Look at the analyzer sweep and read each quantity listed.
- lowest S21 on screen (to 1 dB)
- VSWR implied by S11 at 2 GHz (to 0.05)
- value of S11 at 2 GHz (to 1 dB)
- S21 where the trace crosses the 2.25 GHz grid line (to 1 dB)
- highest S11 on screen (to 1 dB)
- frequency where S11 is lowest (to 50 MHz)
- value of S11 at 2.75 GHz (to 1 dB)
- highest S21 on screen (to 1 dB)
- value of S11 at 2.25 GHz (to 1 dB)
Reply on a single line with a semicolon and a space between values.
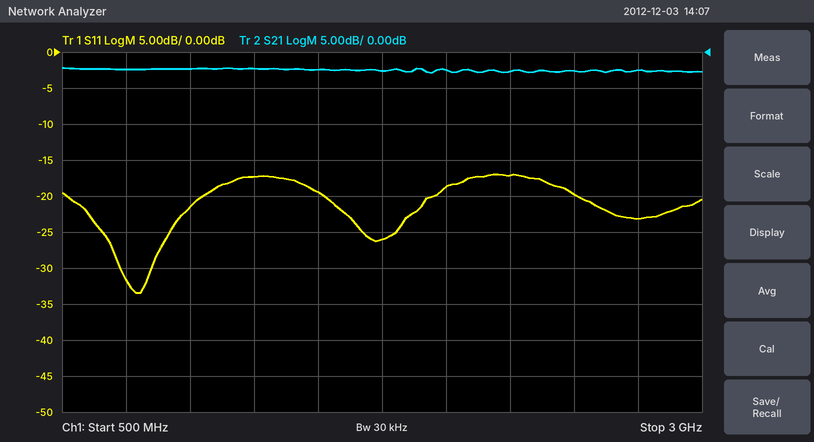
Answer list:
-3 dB; 1.25; -19 dB; -3 dB; -17 dB; 800 MHz; -23 dB; -2 dB; -17 dB
